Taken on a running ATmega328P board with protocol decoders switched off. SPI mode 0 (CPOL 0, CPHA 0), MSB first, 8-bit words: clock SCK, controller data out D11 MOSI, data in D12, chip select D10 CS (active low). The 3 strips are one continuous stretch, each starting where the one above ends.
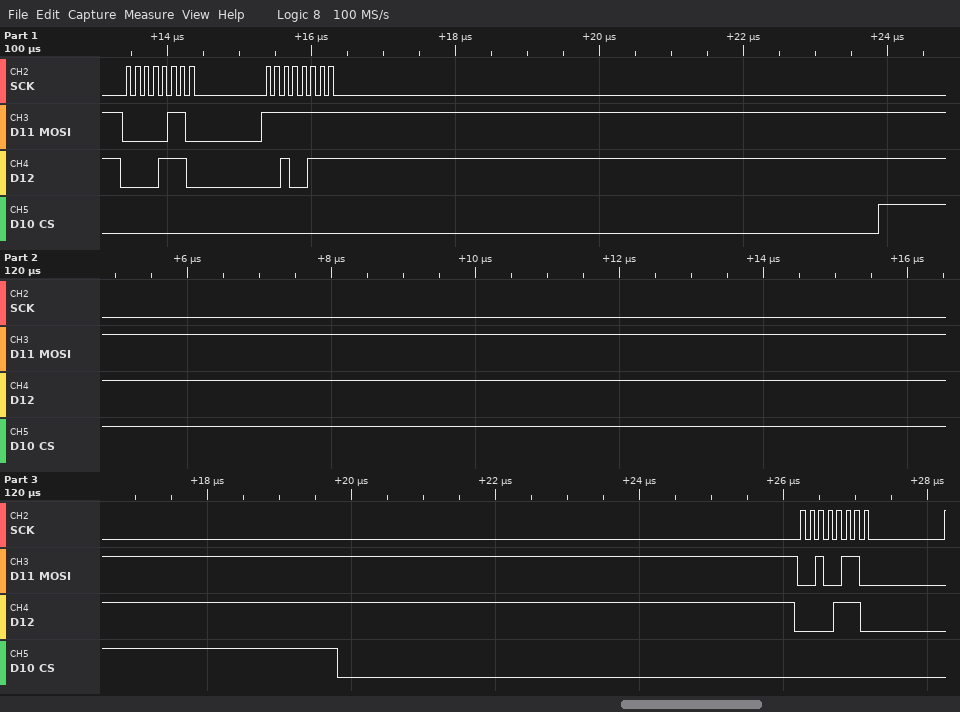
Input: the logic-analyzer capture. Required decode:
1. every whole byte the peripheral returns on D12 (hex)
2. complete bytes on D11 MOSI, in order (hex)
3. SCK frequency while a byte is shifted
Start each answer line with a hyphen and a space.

- 0x0E 0x27 0x0E
- 0x06 0xFF 0x26
- 8 MHz
